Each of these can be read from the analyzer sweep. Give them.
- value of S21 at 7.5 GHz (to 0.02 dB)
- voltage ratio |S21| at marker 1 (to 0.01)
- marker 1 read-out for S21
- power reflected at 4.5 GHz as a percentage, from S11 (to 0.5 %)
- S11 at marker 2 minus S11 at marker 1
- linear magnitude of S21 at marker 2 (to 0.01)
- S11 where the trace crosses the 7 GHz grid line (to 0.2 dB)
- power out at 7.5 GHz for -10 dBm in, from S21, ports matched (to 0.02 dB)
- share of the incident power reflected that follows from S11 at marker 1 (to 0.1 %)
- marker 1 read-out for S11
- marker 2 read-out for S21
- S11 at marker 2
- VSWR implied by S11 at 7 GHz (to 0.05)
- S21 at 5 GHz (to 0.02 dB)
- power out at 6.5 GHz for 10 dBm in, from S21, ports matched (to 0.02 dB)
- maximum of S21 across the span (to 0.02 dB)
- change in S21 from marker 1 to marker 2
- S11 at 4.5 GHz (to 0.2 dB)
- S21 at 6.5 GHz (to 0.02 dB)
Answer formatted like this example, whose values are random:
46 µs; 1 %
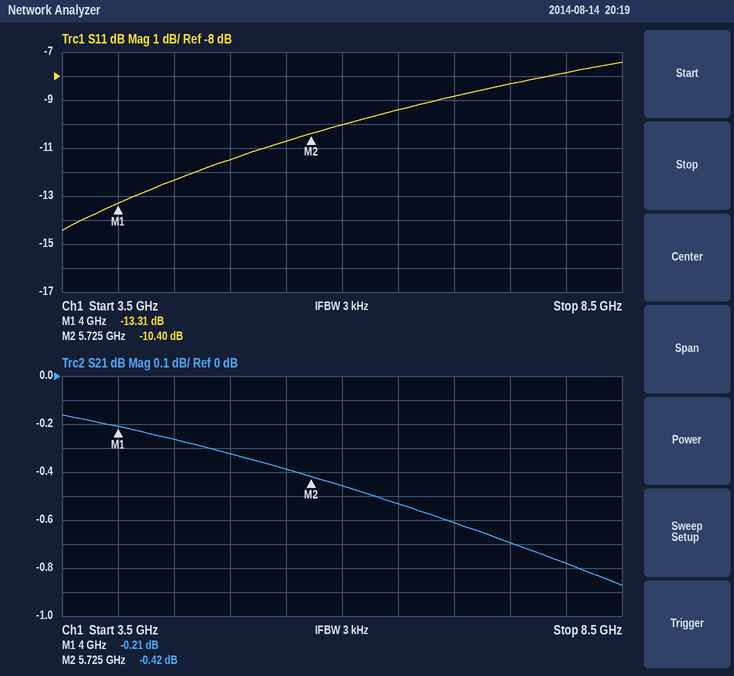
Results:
-0.70 dB; 0.98; -0.21 dB; 6.0 %; 2.91 dB; 0.95; -8.8 dB; -10.70 dBm; 4.7 %; -13.31 dB; -0.42 dB; -10.40 dB; 2.15; -0.32 dB; 9.46 dBm; -0.16 dB; -0.21 dB; -12.4 dB; -0.54 dB
